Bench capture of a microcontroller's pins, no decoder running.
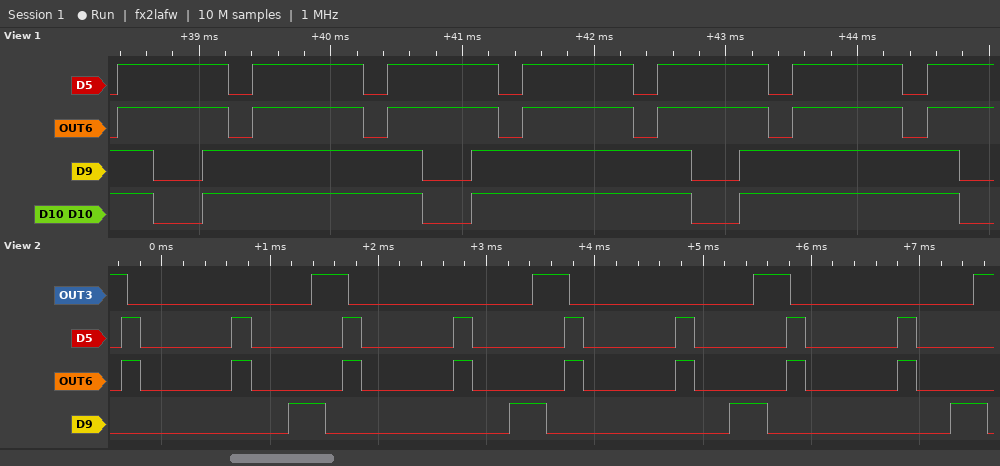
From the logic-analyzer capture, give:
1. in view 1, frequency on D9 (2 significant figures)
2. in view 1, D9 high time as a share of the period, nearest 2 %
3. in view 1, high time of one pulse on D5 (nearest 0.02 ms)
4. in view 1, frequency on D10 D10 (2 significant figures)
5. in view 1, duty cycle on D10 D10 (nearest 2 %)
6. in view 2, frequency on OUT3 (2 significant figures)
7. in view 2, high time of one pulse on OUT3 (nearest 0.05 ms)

490 Hz
82 %
0.84 ms
490 Hz
82 %
490 Hz
0.35 ms
